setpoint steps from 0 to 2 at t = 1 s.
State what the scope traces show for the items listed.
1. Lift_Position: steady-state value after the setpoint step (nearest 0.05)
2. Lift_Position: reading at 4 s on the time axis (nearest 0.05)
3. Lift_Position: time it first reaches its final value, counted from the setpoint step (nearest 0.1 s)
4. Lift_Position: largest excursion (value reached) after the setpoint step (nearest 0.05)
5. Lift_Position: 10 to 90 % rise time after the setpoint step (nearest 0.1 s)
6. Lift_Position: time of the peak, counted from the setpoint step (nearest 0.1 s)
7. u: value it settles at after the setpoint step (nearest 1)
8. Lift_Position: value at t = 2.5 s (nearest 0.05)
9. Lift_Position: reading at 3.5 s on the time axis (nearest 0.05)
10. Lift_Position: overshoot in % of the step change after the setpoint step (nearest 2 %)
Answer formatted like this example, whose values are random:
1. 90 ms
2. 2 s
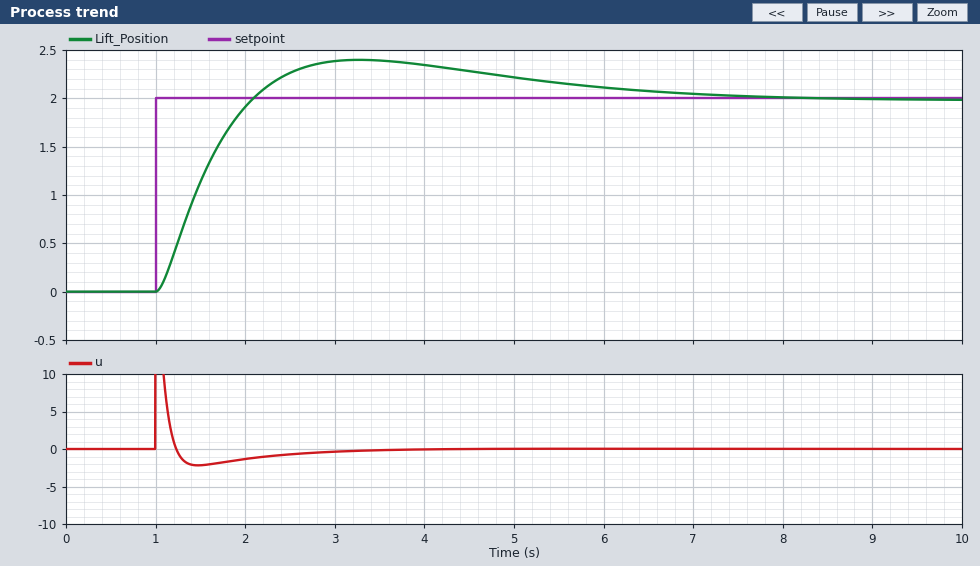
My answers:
1. 2.00
2. 2.35
3. 1.1 s
4. 2.40
5. 0.8 s
6. 2.3 s
7. 0
8. 2.25
9. 2.40
10. 20 %
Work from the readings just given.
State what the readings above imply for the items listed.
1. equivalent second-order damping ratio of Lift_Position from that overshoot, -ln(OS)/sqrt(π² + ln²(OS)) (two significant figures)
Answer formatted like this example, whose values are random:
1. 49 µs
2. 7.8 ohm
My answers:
1. 0.46
